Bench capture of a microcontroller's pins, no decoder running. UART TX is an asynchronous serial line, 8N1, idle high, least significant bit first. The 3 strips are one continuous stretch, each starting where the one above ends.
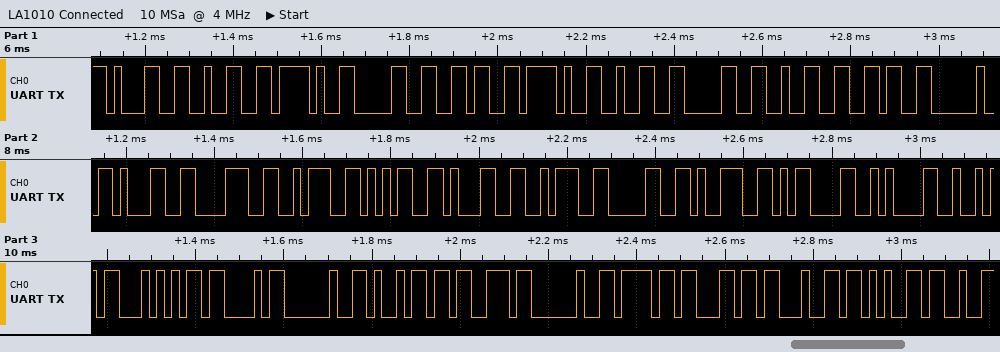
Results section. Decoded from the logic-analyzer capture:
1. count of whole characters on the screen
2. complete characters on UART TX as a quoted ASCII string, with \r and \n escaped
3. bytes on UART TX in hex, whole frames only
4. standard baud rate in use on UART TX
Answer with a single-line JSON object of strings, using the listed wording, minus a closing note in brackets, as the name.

{"count of whole characters on the screen": "32", "complete characters on UART TX as a quoted ASCII string, with \\r and \\n escaped": "\"12/06/2026 18:51:09\\r\\nRTC is olde\"", "bytes on UART TX in hex, whole frames only": "31 32 2F 30 36 2F 32 30 32 36 20 31 38 3A 35 31 3A 30 39 0D 0A 52 54 43 20 69 73 20 6F 6C 64 65", "standard baud rate in use on UART TX": "57600 baud"}
